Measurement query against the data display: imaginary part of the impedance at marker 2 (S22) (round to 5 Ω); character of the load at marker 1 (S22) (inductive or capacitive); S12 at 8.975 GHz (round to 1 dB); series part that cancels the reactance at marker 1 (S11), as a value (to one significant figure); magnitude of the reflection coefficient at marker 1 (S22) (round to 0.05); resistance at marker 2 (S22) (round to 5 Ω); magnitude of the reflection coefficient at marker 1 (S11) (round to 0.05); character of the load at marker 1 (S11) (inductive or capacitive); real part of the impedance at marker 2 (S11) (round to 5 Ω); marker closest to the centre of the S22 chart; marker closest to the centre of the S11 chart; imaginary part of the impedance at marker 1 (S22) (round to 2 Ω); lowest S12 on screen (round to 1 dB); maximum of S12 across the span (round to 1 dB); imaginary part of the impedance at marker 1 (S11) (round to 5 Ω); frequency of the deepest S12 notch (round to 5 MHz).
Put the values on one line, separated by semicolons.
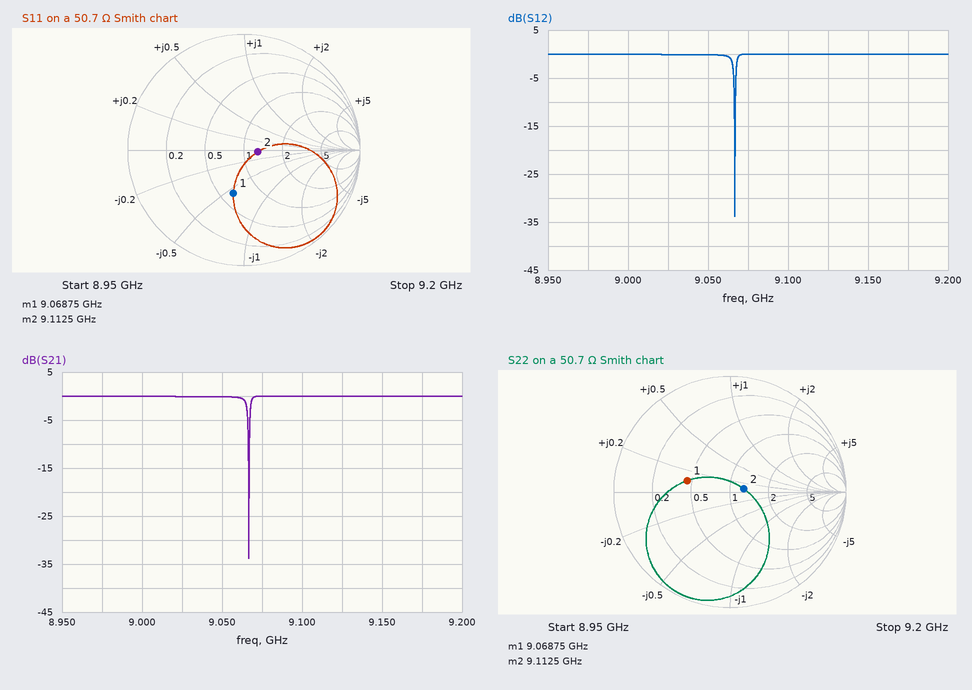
+5 Ω; inductive; 0 dB; 500 pH; 0.40; 65 Ω; 0.40; capacitive; 65 Ω; marker 2; marker 2; +6 Ω; -34 dB; 0 dB; -30 Ω; 9.065 GHz
